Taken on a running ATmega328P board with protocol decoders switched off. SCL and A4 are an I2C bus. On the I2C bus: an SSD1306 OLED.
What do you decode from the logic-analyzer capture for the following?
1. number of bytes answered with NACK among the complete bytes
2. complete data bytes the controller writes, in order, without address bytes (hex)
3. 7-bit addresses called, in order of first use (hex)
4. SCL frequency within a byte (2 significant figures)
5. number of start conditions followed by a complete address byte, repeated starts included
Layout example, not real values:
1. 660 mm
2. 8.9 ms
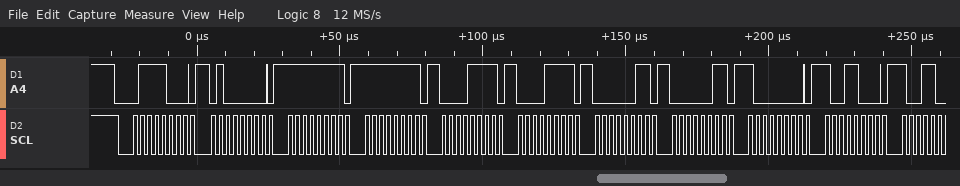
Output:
1. 0
2. 40 FF FF 0F 0F 03 03 80 98
3. 0x3C
4. 400 kHz
5. 1
